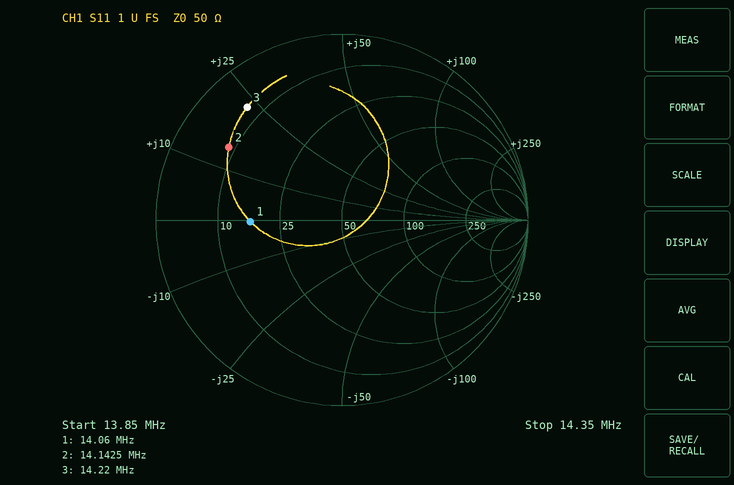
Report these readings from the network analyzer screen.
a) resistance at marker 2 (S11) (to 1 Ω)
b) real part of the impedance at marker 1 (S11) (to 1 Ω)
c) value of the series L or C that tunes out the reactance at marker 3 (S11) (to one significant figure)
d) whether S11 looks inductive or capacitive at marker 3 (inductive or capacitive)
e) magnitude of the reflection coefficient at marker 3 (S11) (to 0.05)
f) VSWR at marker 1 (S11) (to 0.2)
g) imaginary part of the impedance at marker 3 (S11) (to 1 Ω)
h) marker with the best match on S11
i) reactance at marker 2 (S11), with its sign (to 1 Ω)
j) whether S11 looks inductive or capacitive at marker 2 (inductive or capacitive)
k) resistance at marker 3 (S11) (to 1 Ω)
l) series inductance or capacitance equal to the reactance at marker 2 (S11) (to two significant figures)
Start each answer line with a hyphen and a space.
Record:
- 9 Ω
- 17 Ω
- 500 pF
- inductive
- 0.80
- 3.0
- +23 Ω
- marker 1
- +14 Ω
- inductive
- 7 Ω
- 160 nH
